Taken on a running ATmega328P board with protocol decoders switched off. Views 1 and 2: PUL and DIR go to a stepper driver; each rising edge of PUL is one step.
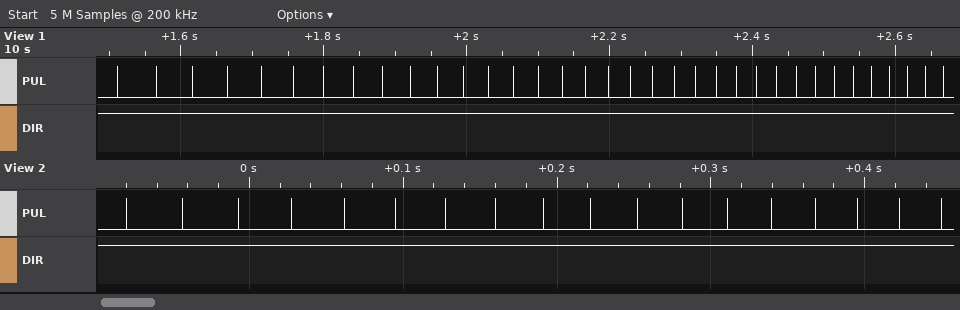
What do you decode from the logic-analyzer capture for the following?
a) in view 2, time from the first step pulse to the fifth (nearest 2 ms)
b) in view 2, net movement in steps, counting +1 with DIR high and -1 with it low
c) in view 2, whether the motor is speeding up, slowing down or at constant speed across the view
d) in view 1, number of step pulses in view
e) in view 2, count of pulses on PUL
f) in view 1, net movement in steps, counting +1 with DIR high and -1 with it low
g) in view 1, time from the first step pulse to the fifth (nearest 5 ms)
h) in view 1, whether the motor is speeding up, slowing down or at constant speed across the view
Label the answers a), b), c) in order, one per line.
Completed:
a) 142 ms
b) +18
c) speeding up
d) 35
e) 18
f) +35
g) 200 ms
h) speeding up
